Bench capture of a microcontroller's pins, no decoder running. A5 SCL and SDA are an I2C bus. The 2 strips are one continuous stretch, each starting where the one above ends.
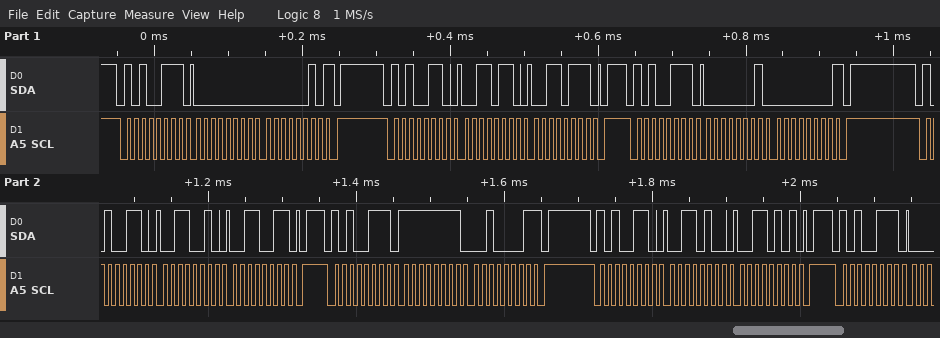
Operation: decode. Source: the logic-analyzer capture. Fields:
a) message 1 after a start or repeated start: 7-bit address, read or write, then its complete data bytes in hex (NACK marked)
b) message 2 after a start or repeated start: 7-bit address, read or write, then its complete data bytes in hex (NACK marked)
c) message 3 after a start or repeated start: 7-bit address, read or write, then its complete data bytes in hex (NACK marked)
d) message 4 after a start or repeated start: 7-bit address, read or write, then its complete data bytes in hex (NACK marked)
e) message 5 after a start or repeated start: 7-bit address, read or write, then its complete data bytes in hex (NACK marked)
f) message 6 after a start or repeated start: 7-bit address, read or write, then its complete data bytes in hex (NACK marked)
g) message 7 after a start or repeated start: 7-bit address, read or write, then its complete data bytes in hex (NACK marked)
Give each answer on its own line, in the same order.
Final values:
0x53 read: 00 02 NACK
0x53 write: 36 37
0x53 read: 01 00 NACK
0x53 write: 32 33
0x53 read: FF 21 NACK
0x53 write: 34 35
0x53 read
